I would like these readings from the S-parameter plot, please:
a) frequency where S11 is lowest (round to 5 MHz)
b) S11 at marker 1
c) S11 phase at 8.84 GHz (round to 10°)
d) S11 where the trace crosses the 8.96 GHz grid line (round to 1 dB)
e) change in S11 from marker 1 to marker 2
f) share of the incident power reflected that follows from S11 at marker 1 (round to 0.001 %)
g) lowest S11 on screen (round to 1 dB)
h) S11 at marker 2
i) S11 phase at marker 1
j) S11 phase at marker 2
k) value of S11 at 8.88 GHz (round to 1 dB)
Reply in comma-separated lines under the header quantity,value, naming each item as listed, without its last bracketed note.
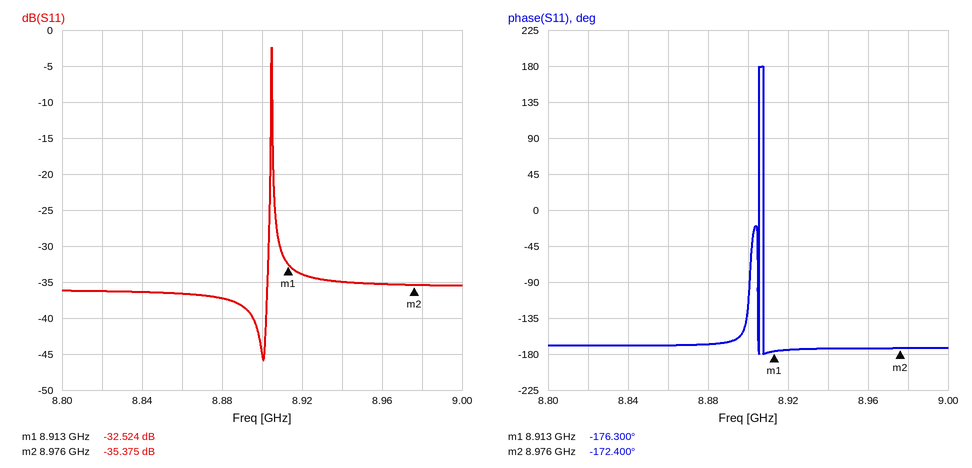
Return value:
quantity,value
frequency where S11 is lowest,8.900 GHz
S11 at marker 1,-32.524 dB
S11 phase at 8.84 GHz,-170°
S11 where the trace crosses the 8.96 GHz grid line,-35 dB
change in S11 from marker 1 to marker 2,-2.851 dB
share of the incident power reflected that follows from S11 at marker 1,0.056 %
lowest S11 on screen,-46 dB
S11 at marker 2,-35.375 dB
S11 phase at marker 1,-176.300°
S11 phase at marker 2,-172.400°
value of S11 at 8.88 GHz,-37 dB
